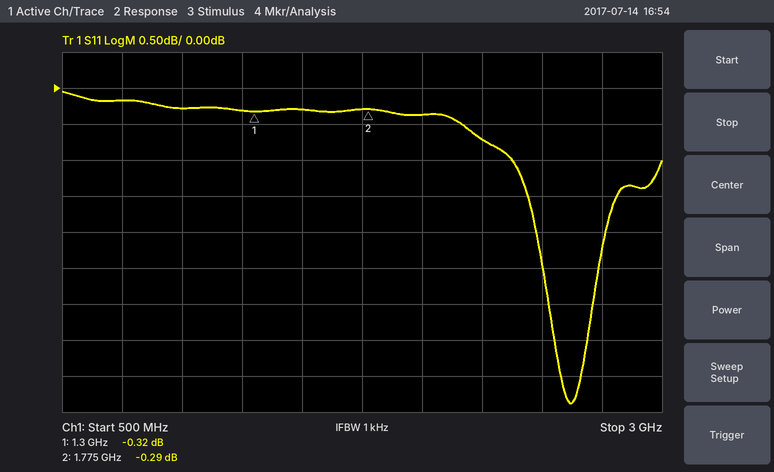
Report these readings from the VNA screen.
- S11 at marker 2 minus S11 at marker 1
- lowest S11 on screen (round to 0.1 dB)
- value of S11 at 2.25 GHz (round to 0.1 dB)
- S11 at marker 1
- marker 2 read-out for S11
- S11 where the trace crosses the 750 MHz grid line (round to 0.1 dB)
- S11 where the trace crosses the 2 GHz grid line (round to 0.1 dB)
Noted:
0.03 dB
-4.4 dB
-0.7 dB
-0.32 dB
-0.29 dB
-0.2 dB
-0.4 dB
